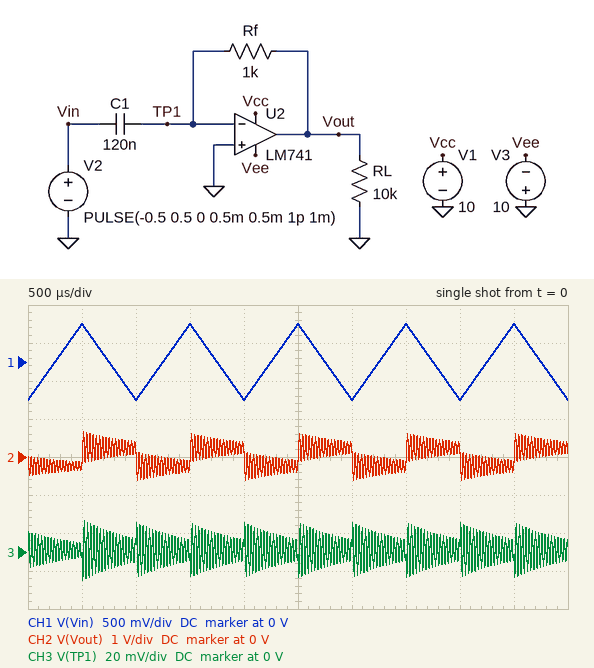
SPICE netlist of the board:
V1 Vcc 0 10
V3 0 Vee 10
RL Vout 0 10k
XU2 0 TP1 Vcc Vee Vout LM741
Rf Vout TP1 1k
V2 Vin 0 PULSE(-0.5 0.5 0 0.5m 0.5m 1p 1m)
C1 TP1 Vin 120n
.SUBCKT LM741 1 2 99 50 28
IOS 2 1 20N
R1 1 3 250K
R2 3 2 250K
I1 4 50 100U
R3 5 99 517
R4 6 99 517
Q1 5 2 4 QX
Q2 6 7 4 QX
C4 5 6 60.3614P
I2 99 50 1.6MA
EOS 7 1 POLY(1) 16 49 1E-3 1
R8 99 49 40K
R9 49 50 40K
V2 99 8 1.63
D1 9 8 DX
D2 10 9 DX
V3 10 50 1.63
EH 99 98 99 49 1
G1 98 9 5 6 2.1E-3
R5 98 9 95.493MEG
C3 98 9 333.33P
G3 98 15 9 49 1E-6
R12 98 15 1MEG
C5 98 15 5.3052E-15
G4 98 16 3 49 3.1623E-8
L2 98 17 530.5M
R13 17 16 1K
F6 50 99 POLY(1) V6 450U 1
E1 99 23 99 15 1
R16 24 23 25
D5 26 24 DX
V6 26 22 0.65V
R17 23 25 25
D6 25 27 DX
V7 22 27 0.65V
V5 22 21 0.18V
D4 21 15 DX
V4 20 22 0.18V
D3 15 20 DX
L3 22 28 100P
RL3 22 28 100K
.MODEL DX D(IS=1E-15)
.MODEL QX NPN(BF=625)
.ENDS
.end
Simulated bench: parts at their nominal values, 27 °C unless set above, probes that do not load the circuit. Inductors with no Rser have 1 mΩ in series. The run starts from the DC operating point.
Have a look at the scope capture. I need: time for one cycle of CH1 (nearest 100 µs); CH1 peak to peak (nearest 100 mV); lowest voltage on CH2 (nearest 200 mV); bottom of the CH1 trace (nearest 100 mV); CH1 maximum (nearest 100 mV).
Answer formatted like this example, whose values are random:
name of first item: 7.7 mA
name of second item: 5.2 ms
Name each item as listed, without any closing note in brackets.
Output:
time for one cycle of CH1: 1.0 ms
CH1 peak to peak: 1.0 V
lowest voltage on CH2: -600 mV
bottom of the CH1 trace: -500 mV
CH1 maximum: 500 mV
